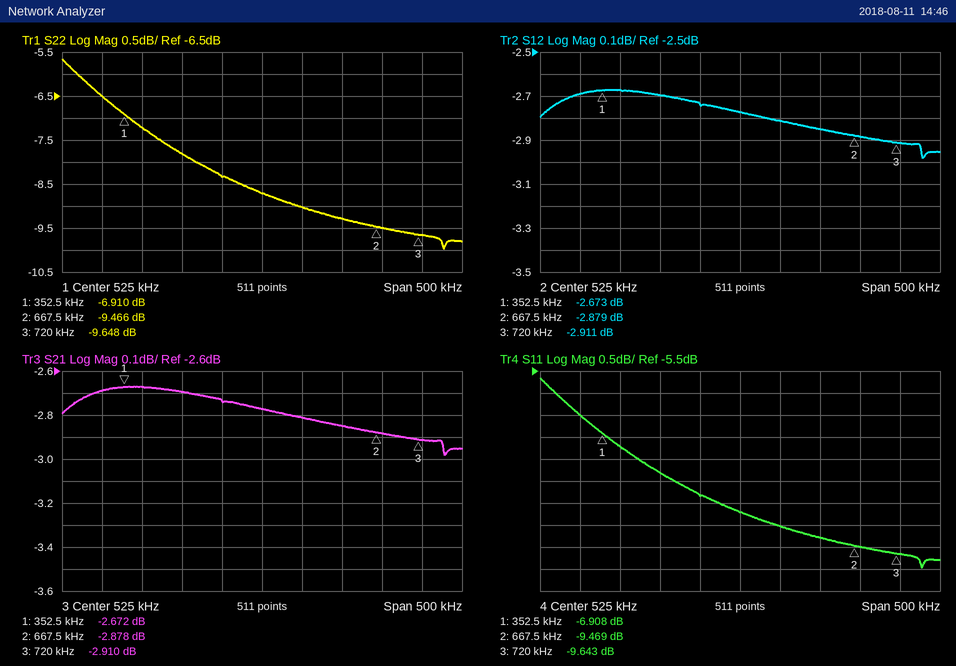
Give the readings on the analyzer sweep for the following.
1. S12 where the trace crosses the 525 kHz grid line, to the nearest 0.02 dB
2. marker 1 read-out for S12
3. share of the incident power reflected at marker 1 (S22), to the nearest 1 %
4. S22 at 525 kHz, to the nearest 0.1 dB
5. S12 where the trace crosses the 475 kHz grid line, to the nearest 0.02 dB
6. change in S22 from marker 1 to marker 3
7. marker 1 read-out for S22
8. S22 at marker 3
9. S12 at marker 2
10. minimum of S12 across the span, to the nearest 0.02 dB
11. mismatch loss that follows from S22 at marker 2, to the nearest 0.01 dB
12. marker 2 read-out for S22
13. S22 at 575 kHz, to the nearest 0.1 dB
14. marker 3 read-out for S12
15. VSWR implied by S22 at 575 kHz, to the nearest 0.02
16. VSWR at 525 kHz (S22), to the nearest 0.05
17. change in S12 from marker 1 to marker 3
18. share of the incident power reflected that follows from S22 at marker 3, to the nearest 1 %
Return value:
-2.78 dB
-2.673 dB
20 %
-8.7 dB
-2.74 dB
-2.738 dB
-6.910 dB
-9.648 dB
-2.879 dB
-2.98 dB
0.52 dB
-9.466 dB
-9.0 dB
-2.911 dB
2.10
2.15
-0.238 dB
11 %
